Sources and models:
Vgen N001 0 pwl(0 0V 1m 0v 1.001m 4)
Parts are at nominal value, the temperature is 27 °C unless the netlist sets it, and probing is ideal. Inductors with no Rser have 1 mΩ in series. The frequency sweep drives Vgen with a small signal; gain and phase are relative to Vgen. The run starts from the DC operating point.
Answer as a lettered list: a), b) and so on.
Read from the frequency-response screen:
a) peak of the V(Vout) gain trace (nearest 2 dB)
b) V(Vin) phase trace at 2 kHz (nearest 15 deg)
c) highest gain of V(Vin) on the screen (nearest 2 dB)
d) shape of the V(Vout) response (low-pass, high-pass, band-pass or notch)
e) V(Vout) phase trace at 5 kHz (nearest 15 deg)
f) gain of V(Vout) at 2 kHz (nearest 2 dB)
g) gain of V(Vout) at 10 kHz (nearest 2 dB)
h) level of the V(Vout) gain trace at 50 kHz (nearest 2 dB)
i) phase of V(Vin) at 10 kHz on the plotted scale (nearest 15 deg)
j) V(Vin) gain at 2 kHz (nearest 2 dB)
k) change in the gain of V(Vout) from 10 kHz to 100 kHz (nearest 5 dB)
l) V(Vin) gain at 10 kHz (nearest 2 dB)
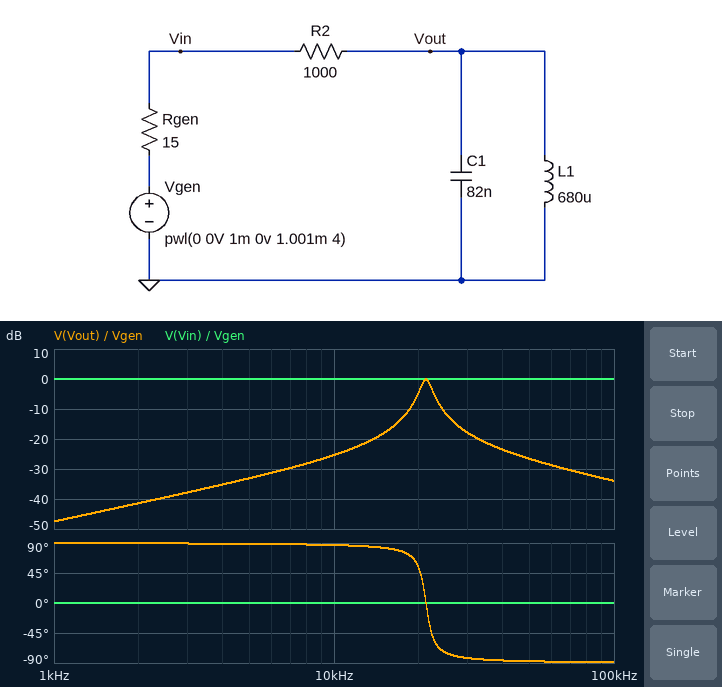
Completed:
a) 0 dB
b) 0 deg
c) 0 dB
d) band-pass
e) 90 deg
f) -42 dB
g) -26 dB
h) -26 dB
i) 0 deg
j) 0 dB
k) -10 dB
l) 0 dB
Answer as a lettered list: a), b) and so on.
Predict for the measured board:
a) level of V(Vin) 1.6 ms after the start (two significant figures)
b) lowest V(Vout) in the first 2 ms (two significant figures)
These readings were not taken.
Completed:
a) 3.9 V
b) -290 mV
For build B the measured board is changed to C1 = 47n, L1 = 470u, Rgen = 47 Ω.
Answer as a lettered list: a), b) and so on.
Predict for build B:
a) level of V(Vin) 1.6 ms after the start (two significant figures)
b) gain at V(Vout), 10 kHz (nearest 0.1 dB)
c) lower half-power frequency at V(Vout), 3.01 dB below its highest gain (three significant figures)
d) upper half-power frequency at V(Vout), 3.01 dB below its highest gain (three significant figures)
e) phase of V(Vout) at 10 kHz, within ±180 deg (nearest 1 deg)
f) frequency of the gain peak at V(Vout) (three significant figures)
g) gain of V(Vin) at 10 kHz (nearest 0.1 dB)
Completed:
a) 3.8 V
b) -30.2 dB
c) 32.3 kHz
d) 35.5 kHz
e) 88 deg
f) 33.9 kHz
g) -0.4 dB
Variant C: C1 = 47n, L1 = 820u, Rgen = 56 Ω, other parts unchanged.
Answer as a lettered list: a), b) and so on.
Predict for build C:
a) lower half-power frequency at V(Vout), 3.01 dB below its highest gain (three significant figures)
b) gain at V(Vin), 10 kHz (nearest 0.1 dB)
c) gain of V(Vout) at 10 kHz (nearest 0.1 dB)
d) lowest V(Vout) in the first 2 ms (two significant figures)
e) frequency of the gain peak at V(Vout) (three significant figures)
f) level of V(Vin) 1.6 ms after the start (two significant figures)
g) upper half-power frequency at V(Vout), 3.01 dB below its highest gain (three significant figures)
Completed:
a) 24.1 kHz
b) -0.5 dB
c) -24.8 dB
d) -370 mV
e) 25.6 kHz
f) 3.8 V
g) 27.3 kHz
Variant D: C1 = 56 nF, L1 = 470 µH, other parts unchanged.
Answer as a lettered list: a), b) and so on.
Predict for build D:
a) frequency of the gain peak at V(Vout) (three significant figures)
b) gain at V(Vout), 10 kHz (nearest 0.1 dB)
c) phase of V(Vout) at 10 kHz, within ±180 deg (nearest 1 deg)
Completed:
a) 31.0 kHz
b) -29.8 dB
c) 88 deg
